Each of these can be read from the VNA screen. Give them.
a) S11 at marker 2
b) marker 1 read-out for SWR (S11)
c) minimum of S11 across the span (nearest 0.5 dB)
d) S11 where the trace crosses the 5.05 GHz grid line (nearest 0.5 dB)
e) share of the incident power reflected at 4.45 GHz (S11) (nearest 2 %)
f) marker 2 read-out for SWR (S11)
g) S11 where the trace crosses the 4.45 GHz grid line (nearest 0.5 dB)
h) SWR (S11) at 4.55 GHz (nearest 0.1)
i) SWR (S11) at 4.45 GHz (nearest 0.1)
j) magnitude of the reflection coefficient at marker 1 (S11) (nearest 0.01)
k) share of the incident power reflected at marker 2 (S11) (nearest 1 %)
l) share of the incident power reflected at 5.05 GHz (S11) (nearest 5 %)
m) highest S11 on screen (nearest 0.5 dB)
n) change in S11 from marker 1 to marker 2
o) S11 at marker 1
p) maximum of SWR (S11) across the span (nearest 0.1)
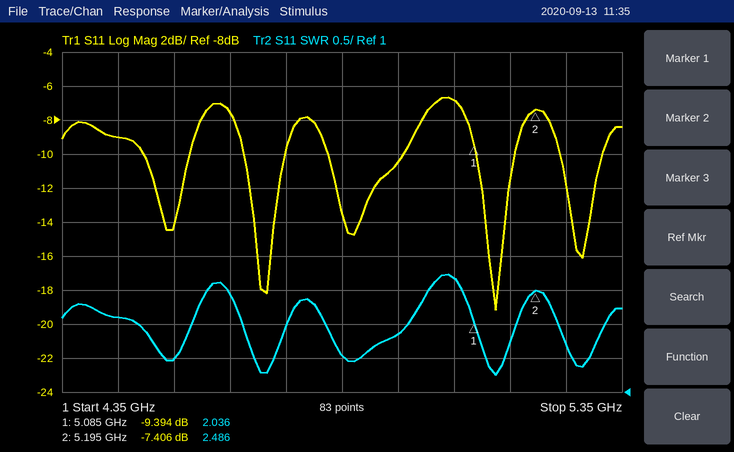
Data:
-7.406 dB
2.036
-19.0 dB
-7.0 dB
12 %
2.486
-9.0 dB
1.5
2.1
0.34
18 %
20 %
-6.5 dB
1.988 dB
-9.394 dB
2.7
